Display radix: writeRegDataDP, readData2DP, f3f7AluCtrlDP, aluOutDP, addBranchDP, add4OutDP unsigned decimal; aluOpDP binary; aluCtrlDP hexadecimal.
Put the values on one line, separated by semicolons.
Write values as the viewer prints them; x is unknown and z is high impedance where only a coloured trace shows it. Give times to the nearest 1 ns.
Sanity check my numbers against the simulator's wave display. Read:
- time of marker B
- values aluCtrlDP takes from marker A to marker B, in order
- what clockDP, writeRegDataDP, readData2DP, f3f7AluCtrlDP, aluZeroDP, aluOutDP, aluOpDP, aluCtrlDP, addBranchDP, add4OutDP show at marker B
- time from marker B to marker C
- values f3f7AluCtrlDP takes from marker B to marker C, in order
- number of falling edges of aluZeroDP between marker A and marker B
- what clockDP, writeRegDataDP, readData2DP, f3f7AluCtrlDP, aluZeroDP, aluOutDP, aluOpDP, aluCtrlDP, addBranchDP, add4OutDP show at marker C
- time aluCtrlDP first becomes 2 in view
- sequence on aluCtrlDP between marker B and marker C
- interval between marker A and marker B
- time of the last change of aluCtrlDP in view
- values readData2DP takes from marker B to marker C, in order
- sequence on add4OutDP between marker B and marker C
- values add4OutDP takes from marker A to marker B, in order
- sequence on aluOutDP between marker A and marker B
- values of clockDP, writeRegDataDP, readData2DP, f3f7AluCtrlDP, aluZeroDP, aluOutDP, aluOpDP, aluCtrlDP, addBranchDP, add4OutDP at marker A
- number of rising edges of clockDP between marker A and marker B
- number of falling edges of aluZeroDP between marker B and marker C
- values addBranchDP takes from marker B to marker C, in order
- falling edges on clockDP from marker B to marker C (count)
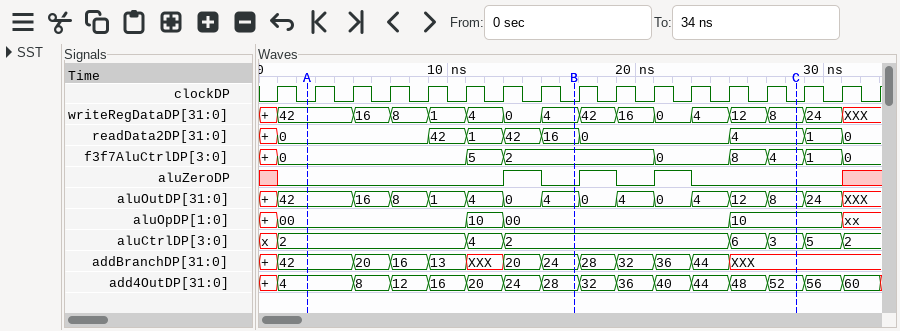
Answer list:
17 ns; 2, 4, 2; clockDP=0, writeRegDataDP=4, readData2DP=16, f3f7AluCtrlDP=2, aluZeroDP=0, aluOutDP=4, aluOpDP=00, aluCtrlDP=2, addBranchDP=24, add4OutDP=28; 12 ns; 2, 0, 8, 4; 1; clockDP=0, writeRegDataDP=8, readData2DP=4, f3f7AluCtrlDP=4, aluZeroDP=0, aluOutDP=8, aluOpDP=10, aluCtrlDP=3, addBranchDP=XXX, add4OutDP=52; 1 ns; 2, 6, 3; 14 ns; 31 ns; 16, 0, 4; 28, 32, 36, 40, 44, 48, 52; 4, 8, 12, 16, 20, 24, 28; 42, 16, 8, 1, 4, 0, 4; clockDP=0, writeRegDataDP=42, readData2DP=0, f3f7AluCtrlDP=0, aluZeroDP=0, aluOutDP=42, aluOpDP=00, aluCtrlDP=2, addBranchDP=42, add4OutDP=4; 7; 2; 24, 28, 32, 36, 44, XXX; 6
